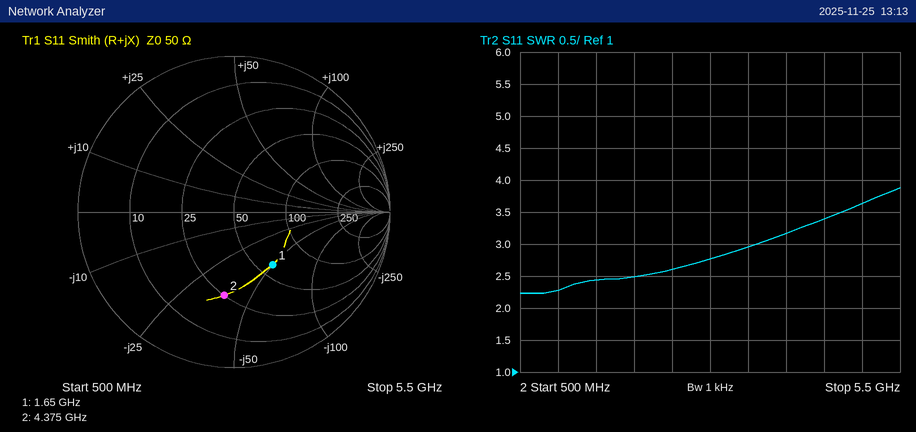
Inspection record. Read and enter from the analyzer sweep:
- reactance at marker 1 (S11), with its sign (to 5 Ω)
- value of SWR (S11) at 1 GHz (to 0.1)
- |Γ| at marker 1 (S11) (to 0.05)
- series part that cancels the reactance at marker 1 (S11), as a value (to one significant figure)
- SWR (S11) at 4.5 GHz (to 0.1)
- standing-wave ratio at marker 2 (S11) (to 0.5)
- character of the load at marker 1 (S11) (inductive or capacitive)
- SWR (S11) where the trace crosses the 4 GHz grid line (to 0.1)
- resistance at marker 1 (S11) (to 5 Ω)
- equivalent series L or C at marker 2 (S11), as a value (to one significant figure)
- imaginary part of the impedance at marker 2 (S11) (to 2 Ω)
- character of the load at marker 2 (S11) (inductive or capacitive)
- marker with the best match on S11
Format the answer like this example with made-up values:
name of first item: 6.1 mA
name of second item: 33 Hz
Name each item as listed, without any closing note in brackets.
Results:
reactance at marker 1 (S11), with its sign: -50 Ω
value of SWR (S11) at 1 GHz: 2.3
|Γ| at marker 1 (S11): 0.40
series part that cancels the reactance at marker 1 (S11), as a value: 5 nH
SWR (S11) at 4.5 GHz: 3.4
standing-wave ratio at marker 2 (S11): 3.5
character of the load at marker 1 (S11): capacitive
SWR (S11) where the trace crosses the 4 GHz grid line: 3.2
resistance at marker 1 (S11): 60 Ω
equivalent series L or C at marker 2 (S11), as a value: 1.0 pF
imaginary part of the impedance at marker 2 (S11): -38 Ω
character of the load at marker 2 (S11): capacitive
marker with the best match on S11: marker 1
